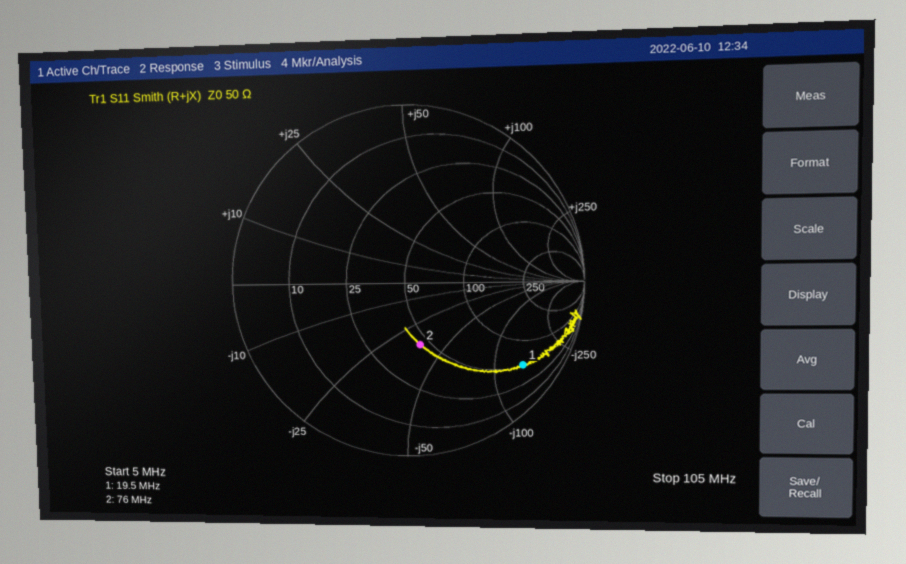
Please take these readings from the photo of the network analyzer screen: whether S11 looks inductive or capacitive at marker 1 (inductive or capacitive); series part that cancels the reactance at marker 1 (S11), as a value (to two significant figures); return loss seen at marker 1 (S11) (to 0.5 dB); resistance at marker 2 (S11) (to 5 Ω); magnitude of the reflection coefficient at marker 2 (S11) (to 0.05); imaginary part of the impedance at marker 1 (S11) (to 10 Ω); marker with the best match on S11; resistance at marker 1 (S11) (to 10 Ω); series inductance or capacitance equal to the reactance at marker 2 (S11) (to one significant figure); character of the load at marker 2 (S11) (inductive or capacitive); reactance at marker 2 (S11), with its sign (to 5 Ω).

capacitive
1.1 µH
2.0 dB
45 Ω
0.35
-140 Ω
marker 2
50 Ω
60 pF
capacitive
-35 Ω
